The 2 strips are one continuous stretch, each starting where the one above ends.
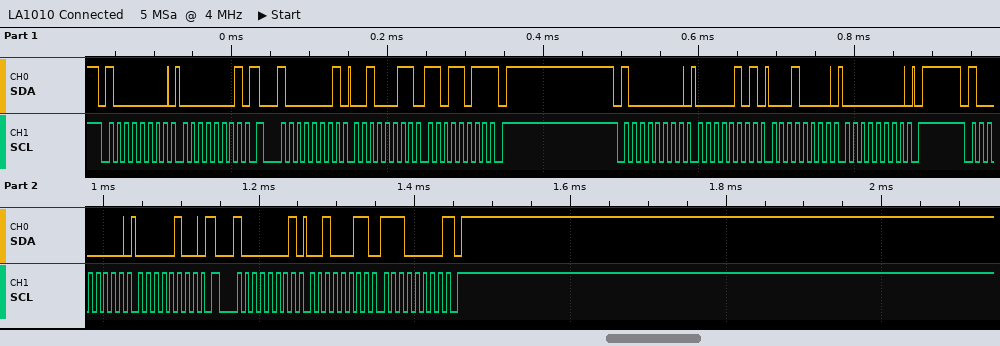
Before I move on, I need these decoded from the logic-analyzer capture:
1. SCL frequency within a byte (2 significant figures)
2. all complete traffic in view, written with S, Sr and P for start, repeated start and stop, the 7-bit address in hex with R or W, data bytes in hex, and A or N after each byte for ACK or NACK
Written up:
100 kHz
S 40W A 01 A Sr 40R A 23 A DB N P S 40W A 05 A 10 A 00 A P S 40W A 04 A Sr 40R A 23 A E0 N P
